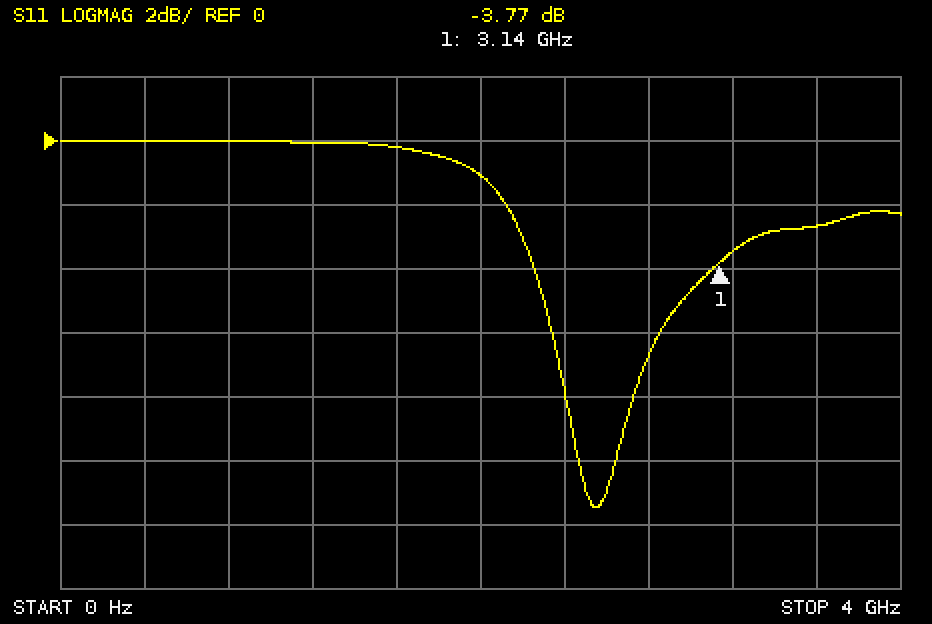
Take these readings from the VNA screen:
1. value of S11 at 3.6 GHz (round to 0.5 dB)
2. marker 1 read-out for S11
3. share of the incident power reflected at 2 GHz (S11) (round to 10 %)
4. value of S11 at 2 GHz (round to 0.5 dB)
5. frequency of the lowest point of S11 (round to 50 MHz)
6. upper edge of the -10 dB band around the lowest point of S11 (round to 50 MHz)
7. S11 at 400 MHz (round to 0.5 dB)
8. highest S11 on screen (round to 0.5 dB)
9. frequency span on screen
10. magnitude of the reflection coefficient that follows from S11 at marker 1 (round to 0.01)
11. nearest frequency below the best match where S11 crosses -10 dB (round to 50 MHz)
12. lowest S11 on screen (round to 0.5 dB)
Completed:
-2.5 dB
-3.77 dB
80 %
-1.0 dB
2.55 GHz
2.65 GHz
0.0 dB
0.0 dB
4 GHz
0.65
2.45 GHz
-11.5 dB
